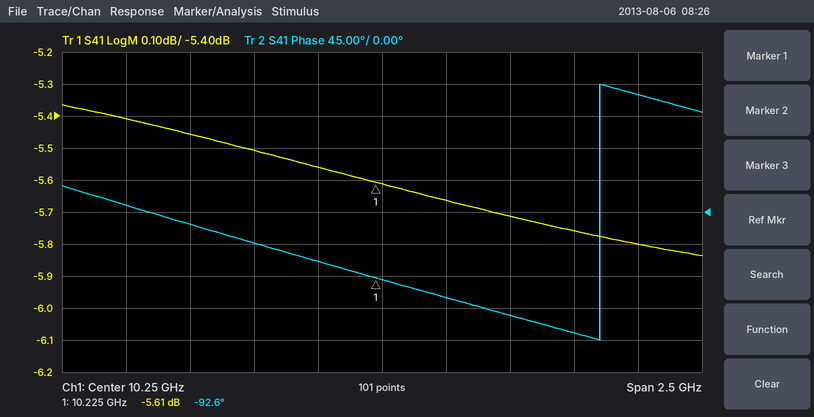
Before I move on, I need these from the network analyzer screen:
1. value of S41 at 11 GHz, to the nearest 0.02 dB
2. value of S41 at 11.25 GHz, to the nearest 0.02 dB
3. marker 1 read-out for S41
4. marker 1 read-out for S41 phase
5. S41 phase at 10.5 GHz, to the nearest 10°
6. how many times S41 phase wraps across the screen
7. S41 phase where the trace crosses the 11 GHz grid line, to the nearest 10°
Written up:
-5.76 dB
-5.80 dB
-5.61 dB
-92.6°
-120°
1
-170°
